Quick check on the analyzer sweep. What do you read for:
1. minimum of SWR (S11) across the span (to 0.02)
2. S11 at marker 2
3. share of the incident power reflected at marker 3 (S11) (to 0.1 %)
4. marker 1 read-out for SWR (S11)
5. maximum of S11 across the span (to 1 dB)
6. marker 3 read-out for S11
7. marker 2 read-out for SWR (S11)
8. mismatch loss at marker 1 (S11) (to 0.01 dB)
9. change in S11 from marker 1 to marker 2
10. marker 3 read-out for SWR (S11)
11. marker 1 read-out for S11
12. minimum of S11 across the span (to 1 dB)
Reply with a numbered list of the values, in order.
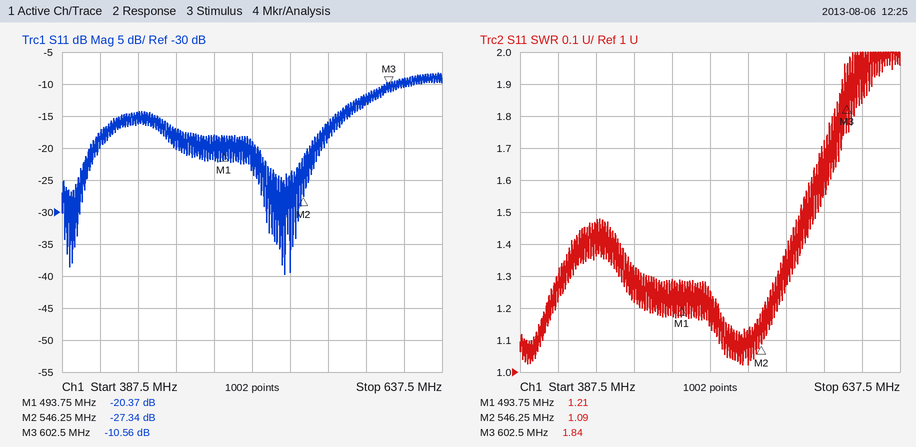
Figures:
1. 1.02
2. -27.34 dB
3. 8.8 %
4. 1.21
5. -8 dB
6. -10.56 dB
7. 1.09
8. 0.04 dB
9. -6.97 dB
10. 1.84
11. -20.37 dB
12. -40 dB
